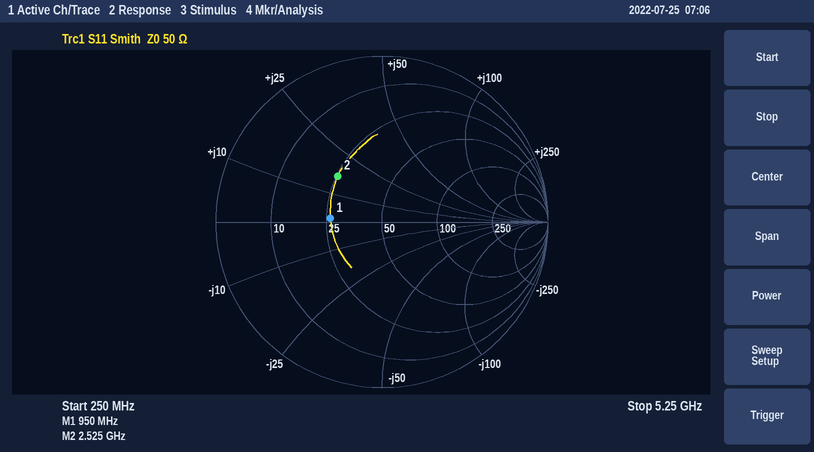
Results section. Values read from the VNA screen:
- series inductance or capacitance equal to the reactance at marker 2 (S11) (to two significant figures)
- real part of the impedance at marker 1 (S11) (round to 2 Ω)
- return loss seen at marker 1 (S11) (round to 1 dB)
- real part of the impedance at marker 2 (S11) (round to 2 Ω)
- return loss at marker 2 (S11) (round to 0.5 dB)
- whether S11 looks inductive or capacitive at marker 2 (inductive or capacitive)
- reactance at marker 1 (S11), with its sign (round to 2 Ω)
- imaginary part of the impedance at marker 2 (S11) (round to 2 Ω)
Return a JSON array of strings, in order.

["1.0 nH", "26 Ω", "10 dB", "26 Ω", "8.5 dB", "inductive", "+2 Ω", "+16 Ω"]
